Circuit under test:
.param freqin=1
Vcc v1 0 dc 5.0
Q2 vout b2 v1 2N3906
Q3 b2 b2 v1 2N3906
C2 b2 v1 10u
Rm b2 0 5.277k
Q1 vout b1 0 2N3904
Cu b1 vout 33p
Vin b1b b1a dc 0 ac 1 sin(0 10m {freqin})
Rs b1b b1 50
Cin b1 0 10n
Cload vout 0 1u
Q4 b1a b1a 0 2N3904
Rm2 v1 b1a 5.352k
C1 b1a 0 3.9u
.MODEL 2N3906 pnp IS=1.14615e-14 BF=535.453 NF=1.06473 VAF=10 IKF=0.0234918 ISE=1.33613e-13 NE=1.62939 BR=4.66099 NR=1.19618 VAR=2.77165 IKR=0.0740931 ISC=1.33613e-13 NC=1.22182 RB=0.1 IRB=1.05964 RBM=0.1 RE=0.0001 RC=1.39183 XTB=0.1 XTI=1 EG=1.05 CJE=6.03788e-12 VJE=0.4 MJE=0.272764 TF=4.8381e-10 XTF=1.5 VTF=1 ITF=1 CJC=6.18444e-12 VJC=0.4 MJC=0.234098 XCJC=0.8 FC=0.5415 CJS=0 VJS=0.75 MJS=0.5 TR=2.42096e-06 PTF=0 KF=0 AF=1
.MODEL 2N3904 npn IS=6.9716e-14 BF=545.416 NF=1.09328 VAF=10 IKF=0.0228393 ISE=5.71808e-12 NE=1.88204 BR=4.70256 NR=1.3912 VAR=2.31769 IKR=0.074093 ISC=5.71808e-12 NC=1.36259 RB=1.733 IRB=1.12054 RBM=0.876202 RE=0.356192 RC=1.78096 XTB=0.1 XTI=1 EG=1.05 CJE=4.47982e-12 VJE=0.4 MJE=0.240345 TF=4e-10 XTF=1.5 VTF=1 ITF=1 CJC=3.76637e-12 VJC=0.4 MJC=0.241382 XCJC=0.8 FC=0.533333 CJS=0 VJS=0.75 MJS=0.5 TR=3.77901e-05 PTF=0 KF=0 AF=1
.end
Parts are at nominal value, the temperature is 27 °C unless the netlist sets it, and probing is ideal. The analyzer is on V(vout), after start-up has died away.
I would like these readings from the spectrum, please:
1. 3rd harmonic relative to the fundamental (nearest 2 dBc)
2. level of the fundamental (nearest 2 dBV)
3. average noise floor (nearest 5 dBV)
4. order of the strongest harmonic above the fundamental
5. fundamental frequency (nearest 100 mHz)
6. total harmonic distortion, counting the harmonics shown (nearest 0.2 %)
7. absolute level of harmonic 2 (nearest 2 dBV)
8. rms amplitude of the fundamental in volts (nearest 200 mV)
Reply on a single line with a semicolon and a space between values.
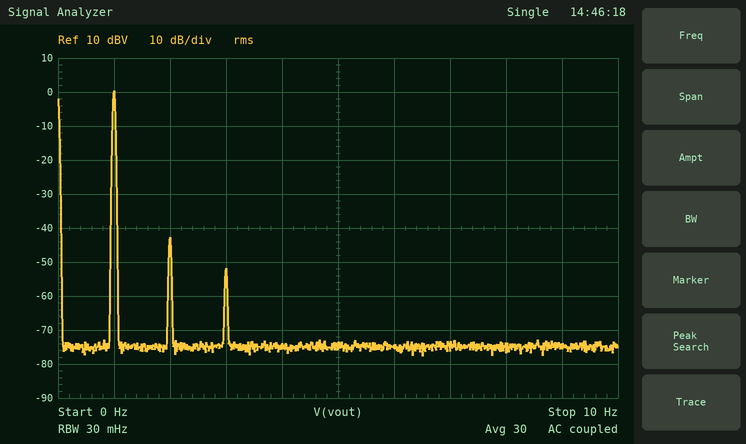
-52 dBc; 0 dBV; -75 dBV; 2; 1.0 Hz; 0.8 %; -42 dBV; 1.0 V
